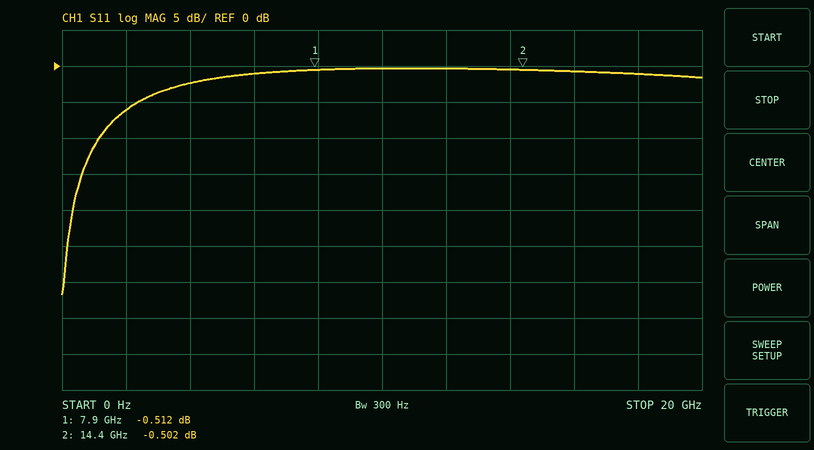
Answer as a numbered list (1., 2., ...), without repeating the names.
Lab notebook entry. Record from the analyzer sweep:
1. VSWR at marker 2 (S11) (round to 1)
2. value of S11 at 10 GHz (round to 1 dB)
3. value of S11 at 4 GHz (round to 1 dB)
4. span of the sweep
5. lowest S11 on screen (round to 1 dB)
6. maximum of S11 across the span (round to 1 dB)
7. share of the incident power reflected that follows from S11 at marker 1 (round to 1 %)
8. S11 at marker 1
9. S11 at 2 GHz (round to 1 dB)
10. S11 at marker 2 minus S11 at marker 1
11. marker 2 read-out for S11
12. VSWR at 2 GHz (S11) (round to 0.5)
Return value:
1. 35
2. 0 dB
3. -2 dB
4. 20 GHz
5. -32 dB
6. 0 dB
7. 89 %
8. -0.512 dB
9. -6 dB
10. 0.010 dB
11. -0.502 dB
12. 3.0
